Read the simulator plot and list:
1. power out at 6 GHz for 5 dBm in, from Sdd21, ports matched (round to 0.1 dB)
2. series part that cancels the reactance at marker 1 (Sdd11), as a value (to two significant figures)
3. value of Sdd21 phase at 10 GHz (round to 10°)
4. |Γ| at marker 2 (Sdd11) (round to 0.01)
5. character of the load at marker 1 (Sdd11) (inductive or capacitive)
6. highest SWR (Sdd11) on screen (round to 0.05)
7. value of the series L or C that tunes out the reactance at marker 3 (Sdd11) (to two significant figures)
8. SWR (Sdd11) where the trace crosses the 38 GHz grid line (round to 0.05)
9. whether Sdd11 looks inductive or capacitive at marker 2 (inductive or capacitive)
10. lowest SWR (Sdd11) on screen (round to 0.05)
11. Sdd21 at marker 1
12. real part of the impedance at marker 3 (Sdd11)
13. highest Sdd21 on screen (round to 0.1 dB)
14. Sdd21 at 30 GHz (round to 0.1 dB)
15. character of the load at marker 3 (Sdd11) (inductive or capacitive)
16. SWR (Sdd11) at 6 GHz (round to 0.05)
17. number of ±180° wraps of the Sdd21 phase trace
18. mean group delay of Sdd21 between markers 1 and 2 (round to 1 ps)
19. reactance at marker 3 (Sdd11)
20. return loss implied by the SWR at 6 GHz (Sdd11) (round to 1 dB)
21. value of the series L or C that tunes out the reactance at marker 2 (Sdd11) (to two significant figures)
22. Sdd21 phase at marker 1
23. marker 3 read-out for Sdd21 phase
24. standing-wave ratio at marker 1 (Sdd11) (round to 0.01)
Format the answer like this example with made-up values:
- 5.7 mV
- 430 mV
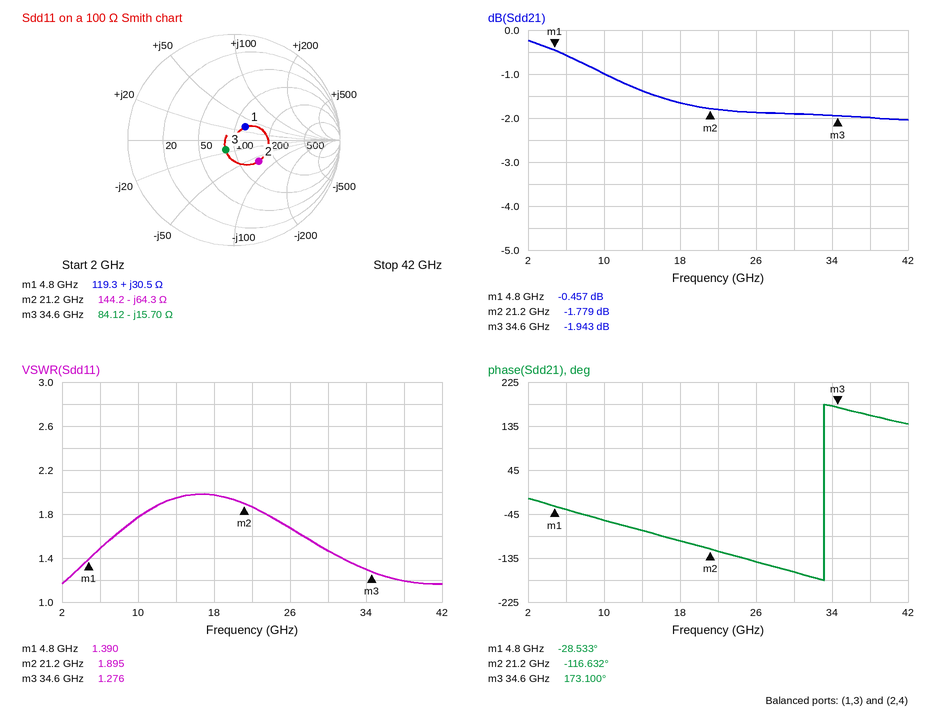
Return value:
- 4.4 dBm
- 1.1 pF
- -60°
- 0.31
- inductive
- 2.00
- 72 pH
- 1.20
- capacitive
- 1.15
- -0.457 dB
- 84.12 Ω
- -0.2 dB
- -1.9 dB
- capacitive
- 1.50
- 1
- 15 ps
- -15.70 Ω
- 14 dB
- 480 pH
- -28.533°
- 173.100°
- 1.39
